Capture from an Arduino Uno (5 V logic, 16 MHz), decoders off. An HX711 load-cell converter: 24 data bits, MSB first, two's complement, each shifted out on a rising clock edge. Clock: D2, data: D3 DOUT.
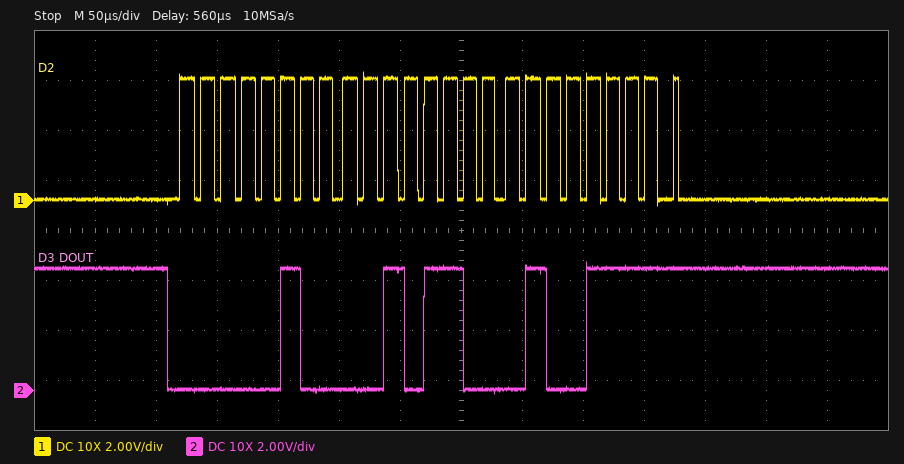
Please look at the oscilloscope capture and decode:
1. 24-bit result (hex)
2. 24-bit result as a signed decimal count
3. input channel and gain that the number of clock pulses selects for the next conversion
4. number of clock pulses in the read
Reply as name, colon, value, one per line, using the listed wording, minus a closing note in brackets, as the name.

24-bit result: 0x042C4F
24-bit result as a signed decimal count: 273487
input channel and gain that the number of clock pulses selects for the next conversion: channel A, gain 128
number of clock pulses in the read: 25
